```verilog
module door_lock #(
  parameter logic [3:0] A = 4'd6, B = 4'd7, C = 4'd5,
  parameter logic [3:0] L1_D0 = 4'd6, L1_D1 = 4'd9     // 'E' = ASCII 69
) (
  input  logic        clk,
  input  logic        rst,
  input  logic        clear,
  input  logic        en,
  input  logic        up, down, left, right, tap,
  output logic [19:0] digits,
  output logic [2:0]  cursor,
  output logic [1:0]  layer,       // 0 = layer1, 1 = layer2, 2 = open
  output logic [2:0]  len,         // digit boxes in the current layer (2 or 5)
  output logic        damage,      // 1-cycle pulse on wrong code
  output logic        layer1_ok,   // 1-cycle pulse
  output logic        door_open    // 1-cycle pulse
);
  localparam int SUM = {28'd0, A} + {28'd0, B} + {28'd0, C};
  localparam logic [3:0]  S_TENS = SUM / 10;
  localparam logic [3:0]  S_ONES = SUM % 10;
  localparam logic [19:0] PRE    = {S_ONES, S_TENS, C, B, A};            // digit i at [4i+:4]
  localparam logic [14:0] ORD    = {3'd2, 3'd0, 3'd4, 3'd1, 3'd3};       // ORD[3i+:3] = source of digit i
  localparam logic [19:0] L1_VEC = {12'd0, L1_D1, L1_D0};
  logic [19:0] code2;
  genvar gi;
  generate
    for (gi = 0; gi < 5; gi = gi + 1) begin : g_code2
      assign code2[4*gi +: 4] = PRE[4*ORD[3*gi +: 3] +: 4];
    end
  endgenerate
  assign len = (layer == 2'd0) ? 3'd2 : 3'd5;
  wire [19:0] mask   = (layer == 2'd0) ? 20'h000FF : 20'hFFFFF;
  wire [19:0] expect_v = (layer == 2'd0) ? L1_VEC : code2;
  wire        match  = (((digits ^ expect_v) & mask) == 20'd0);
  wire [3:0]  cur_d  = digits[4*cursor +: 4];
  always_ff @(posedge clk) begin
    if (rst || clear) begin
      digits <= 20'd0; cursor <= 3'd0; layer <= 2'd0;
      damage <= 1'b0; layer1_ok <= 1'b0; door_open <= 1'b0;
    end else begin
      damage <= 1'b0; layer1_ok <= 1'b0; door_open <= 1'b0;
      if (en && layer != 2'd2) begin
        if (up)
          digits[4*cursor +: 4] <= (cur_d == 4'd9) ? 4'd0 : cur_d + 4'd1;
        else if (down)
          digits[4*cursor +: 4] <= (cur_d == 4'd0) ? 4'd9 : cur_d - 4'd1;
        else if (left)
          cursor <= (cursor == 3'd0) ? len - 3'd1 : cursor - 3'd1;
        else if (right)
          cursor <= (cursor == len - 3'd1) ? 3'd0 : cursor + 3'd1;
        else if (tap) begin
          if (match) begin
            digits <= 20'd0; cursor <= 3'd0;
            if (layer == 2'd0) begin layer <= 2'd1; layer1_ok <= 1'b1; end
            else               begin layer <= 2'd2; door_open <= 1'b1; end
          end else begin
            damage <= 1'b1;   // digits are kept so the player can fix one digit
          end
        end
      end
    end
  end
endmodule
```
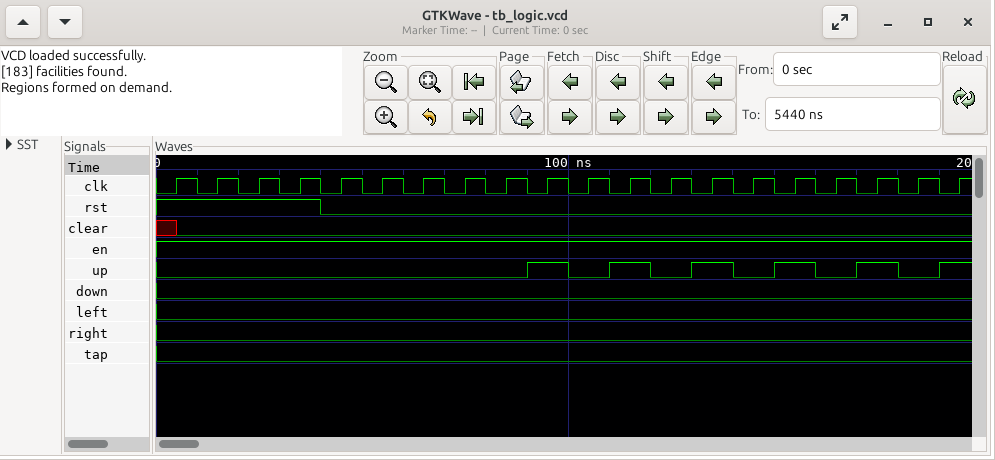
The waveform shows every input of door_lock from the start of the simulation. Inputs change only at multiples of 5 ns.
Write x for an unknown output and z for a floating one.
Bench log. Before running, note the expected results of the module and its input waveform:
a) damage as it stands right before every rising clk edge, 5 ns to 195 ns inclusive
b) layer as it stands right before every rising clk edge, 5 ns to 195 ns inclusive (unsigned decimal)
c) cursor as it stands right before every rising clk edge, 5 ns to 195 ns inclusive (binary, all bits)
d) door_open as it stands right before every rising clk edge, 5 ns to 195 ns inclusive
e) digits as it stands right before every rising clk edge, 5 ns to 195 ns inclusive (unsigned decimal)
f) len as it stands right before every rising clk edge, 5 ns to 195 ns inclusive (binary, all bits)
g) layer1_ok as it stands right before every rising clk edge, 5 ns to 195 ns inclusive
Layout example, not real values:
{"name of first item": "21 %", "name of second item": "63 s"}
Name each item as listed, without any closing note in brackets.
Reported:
{"damage as it stands right before every rising clk edge, 5 ns to 195 ns inclusive": "x 0 0 0 0 0 0 0 0 0 0 0 0 0 0 0 0 0 0 0", "layer as it stands right before every rising clk edge, 5 ns to 195 ns inclusive": "x, 0, 0, 0, 0, 0, 0, 0, 0, 0, 0, 0, 0, 0, 0, 0, 0, 0, 0, 0", "cursor as it stands right before every rising clk edge, 5 ns to 195 ns inclusive": "x, 000, 000, 000, 000, 000, 000, 000, 000, 000, 000, 000, 000, 000, 000, 000, 000, 000, 000, 000", "door_open as it stands right before every rising clk edge, 5 ns to 195 ns inclusive": "x 0 0 0 0 0 0 0 0 0 0 0 0 0 0 0 0 0 0 0", "digits as it stands right before every rising clk edge, 5 ns to 195 ns inclusive": "x, 0, 0, 0, 0, 0, 0, 0, 0, 0, 1, 1, 2, 2, 3, 3, 4, 4, 5, 5", "len as it stands right before every rising clk edge, 5 ns to 195 ns inclusive": "x, 010, 010, 010, 010, 010, 010, 010, 010, 010, 010, 010, 010, 010, 010, 010, 010, 010, 010, 010", "layer1_ok as it stands right before every rising clk edge, 5 ns to 195 ns inclusive": "x 0 0 0 0 0 0 0 0 0 0 0 0 0 0 0 0 0 0 0"}
